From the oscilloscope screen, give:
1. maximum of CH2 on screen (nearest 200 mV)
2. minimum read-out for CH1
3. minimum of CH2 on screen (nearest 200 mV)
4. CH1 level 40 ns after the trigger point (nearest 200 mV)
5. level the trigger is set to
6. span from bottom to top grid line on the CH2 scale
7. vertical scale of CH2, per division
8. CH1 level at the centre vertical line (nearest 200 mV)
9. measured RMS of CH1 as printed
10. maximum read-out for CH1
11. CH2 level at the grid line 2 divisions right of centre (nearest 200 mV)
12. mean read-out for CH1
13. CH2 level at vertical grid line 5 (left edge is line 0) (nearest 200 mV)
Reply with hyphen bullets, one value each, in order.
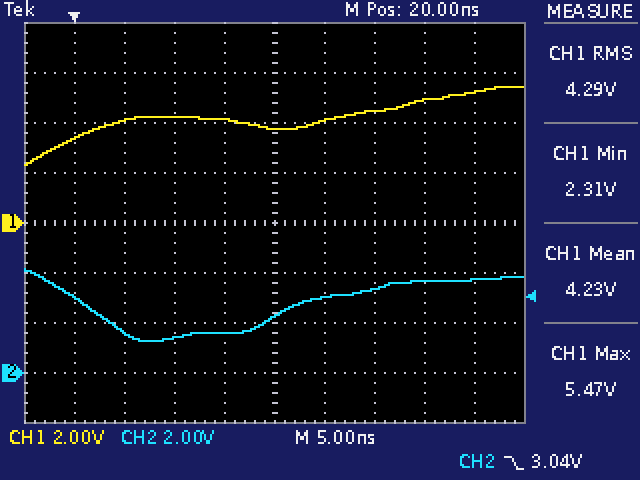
- 4.2 V
- 2.31 V
- 1.2 V
- 5.2 V
- 3.04 V
- 16 V
- 2 V
- 3.8 V
- 4.29 V
- 5.47 V
- 3.4 V
- 4.23 V
- 2.2 V
